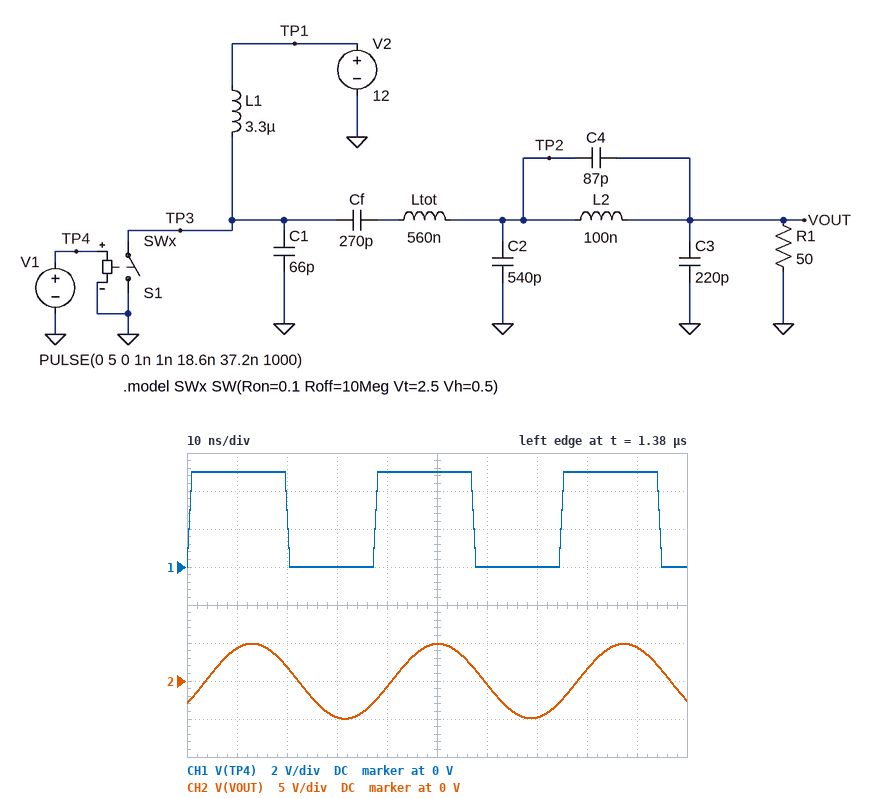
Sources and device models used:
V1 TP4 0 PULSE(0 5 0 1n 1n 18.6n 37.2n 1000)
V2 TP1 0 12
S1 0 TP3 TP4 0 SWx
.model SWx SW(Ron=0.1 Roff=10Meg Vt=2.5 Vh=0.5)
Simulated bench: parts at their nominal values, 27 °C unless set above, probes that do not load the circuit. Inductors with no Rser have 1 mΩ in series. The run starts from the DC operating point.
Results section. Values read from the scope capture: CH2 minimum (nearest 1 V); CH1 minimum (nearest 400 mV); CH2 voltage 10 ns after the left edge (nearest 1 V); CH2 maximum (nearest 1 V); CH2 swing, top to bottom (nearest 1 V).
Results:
-5 V
0 V
4 V
5 V
10 V
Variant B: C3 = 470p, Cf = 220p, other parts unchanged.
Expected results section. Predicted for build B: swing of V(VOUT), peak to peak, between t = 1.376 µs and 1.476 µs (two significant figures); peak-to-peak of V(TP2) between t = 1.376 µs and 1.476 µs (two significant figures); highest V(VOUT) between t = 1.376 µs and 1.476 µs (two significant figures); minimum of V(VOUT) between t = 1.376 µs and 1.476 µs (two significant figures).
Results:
23 V
20 V
11 V
-11 V
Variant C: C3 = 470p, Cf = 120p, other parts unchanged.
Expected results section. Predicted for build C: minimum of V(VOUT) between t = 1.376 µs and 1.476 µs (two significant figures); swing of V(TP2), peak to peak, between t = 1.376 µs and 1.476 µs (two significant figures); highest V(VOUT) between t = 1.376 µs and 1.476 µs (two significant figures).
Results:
-15 V
27 V
15 V
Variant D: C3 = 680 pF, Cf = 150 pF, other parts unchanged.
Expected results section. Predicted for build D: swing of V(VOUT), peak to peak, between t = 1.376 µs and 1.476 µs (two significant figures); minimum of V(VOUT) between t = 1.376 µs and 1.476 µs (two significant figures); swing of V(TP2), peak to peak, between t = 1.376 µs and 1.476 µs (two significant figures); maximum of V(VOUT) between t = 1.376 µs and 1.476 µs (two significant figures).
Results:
54 V
-27 V
88 V
27 V
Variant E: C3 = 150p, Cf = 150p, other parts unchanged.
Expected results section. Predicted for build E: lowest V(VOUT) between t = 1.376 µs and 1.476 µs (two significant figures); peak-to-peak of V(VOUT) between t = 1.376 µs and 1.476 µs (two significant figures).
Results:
-6.0 V
12 V
